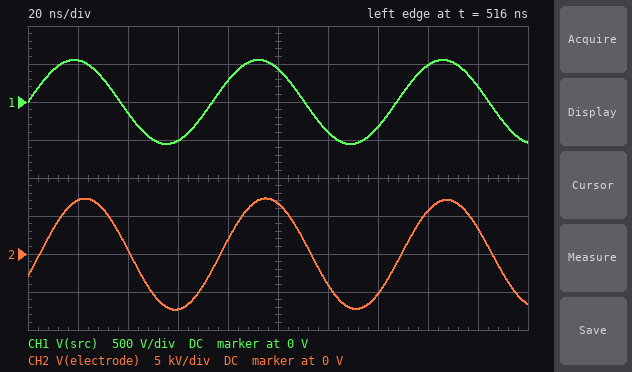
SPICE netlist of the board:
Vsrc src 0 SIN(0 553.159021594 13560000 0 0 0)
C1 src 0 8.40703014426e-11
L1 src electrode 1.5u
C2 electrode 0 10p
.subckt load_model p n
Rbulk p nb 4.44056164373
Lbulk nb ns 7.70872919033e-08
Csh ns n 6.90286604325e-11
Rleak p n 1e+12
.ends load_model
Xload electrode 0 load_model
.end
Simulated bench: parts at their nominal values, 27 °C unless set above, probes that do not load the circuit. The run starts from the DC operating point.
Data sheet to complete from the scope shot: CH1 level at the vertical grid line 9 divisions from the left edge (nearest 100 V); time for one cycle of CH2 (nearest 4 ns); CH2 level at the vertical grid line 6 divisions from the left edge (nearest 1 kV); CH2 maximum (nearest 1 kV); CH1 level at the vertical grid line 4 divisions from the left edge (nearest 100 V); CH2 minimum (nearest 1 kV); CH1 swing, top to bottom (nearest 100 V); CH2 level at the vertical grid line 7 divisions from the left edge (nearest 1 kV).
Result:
200 V
72 ns
-4 kV
7 kV
300 V
-7 kV
1.1 kV
-5 kV
